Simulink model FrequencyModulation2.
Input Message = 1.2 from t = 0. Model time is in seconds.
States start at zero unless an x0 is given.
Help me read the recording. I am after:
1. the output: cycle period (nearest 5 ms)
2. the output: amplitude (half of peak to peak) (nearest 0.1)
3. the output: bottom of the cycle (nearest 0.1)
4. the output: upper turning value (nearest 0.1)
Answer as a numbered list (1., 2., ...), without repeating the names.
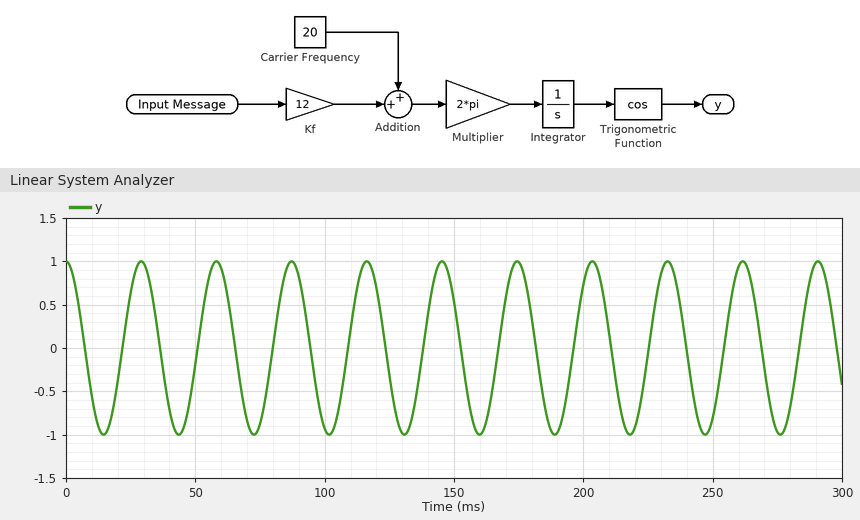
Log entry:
1. 30 ms
2. 1.0
3. -1.0
4. 1.0
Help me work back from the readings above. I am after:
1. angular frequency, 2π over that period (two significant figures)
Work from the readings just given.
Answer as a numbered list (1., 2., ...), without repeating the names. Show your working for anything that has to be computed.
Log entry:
1. 2π / 30 = 0.21 rad/ms
